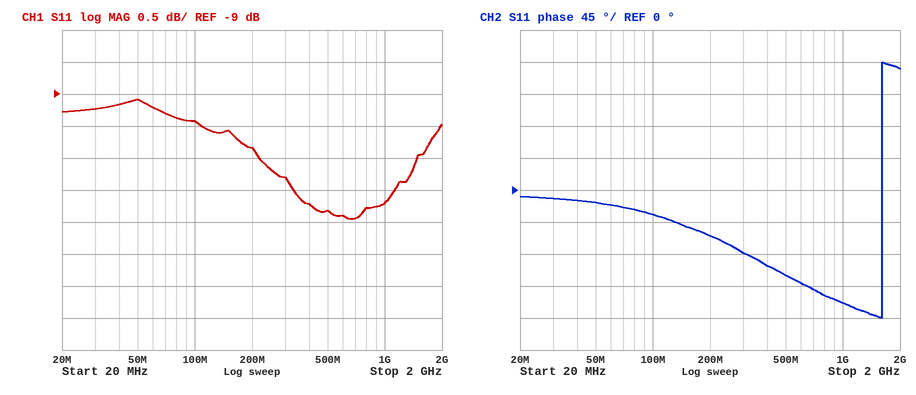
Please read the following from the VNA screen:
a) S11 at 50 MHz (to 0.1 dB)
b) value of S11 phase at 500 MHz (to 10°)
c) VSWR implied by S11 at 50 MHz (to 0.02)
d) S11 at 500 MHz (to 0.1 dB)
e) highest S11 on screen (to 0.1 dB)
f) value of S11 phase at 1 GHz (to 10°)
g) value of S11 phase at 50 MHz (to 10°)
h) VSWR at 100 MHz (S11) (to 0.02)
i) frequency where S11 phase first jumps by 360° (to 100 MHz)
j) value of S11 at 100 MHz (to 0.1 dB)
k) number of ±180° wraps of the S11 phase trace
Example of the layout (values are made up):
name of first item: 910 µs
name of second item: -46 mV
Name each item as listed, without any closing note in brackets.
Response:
S11 at 50 MHz: -9.1 dB
value of S11 phase at 500 MHz: -120°
VSWR implied by S11 at 50 MHz: 2.08
S11 at 500 MHz: -10.8 dB
highest S11 on screen: -9.1 dB
value of S11 phase at 1 GHz: -160°
value of S11 phase at 50 MHz: -20°
VSWR at 100 MHz (S11): 2.02
frequency where S11 phase first jumps by 360°: 1.6 GHz
value of S11 at 100 MHz: -9.4 dB
number of ±180° wraps of the S11 phase trace: 1
